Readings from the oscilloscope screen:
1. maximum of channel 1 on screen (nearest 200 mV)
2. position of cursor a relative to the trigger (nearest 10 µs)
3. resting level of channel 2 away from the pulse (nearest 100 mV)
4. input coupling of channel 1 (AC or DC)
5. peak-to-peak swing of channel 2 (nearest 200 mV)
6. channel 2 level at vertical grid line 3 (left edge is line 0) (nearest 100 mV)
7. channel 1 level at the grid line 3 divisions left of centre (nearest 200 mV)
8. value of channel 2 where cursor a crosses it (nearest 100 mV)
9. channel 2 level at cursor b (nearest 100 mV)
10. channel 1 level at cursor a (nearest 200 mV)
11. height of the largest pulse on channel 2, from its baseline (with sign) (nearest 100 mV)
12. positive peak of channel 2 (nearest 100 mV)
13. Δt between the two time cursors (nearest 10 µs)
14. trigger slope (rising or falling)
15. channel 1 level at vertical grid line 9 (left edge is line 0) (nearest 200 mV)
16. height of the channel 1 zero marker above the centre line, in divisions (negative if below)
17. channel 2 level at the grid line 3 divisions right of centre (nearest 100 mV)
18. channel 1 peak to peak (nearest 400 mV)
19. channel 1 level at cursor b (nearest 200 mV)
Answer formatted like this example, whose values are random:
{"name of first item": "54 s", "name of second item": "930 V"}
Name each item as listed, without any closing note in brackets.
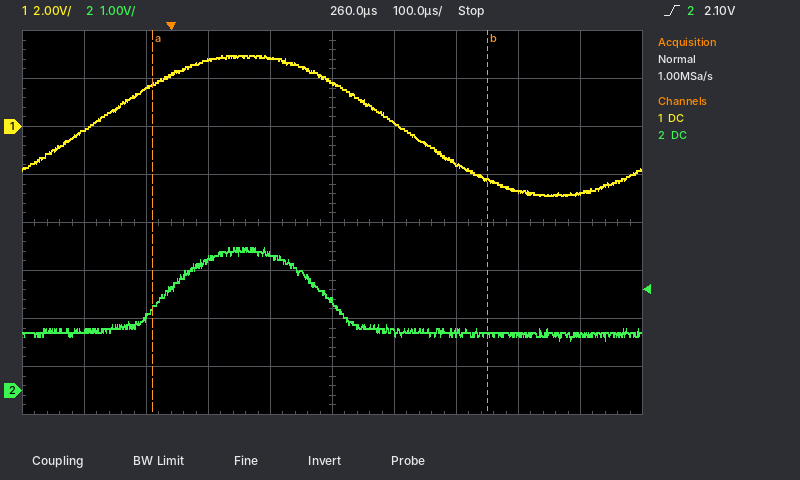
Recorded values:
{"maximum of channel 1 on screen": "3.0 V", "position of cursor a relative to the trigger": "-30 µs", "resting level of channel 2 away from the pulse": "1.2 V", "input coupling of channel 1": "DC", "peak-to-peak swing of channel 2": "2.0 V", "channel 2 level at vertical grid line 3 (left edge is line 0)": "2.7 V", "channel 1 level at the grid line 3 divisions left of centre": "1.6 V", "value of channel 2 where cursor a crosses it": "1.7 V", "channel 2 level at cursor b": "1.2 V", "channel 1 level at cursor a": "1.8 V", "height of the largest pulse on channel 2, from its baseline (with sign)": "+1.8 V", "positive peak of channel 2": "3.0 V", "Δt between the two time cursors": "540 µs", "trigger slope": "rising", "channel 1 level at vertical grid line 9 (left edge is line 0)": "-2.8 V", "height of the channel 1 zero marker above the centre line, in divisions": "+2.0 div", "channel 2 level at the grid line 3 divisions right of centre": "1.2 V", "channel 1 peak to peak": "6.0 V", "channel 1 level at cursor b": "-2.2 V"}
